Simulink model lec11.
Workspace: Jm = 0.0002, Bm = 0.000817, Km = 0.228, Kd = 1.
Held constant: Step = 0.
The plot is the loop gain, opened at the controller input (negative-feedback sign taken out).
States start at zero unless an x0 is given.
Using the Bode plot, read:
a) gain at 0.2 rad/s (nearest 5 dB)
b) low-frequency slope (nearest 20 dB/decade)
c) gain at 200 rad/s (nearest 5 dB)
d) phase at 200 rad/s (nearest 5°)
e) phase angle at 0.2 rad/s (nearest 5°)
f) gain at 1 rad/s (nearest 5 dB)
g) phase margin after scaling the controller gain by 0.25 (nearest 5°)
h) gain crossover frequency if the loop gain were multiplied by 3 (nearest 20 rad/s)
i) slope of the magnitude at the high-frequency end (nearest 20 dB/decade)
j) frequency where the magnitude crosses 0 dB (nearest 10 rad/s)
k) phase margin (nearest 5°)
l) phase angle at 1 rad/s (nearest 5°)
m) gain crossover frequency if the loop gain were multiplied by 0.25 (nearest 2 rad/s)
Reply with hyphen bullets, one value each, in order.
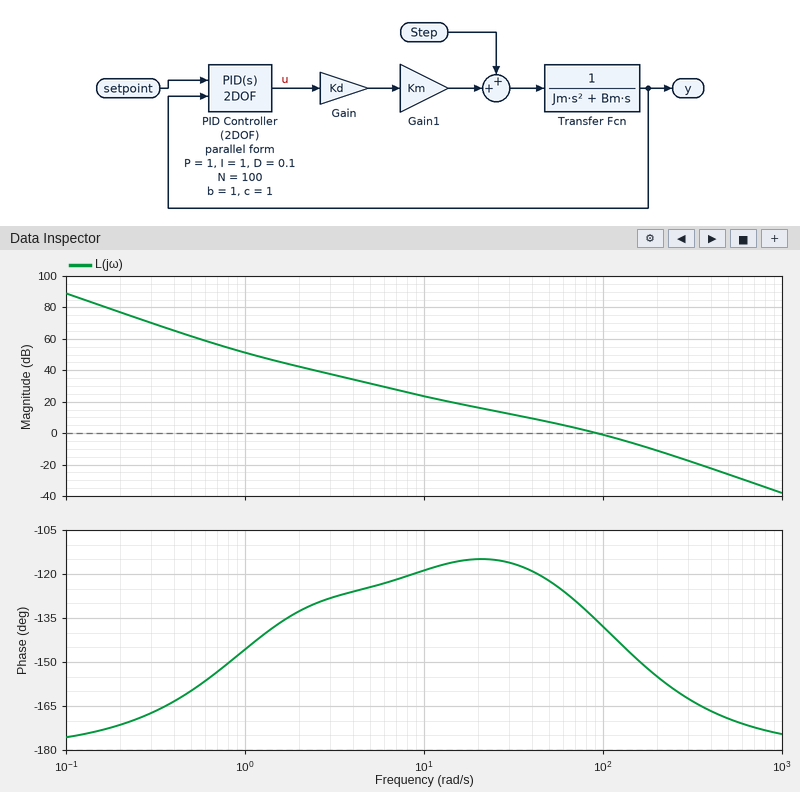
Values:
- 75 dB
- -40 dB/decade
- -10 dB
- -155°
- -170°
- 50 dB
- 65°
- 180 rad/s
- -40 dB/decade
- 90 rad/s
- 45°
- -145°
- 30 rad/s
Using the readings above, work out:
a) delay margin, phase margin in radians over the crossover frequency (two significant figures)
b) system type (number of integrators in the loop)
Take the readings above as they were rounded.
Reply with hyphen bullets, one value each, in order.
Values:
- 0.0087 s
- 2
